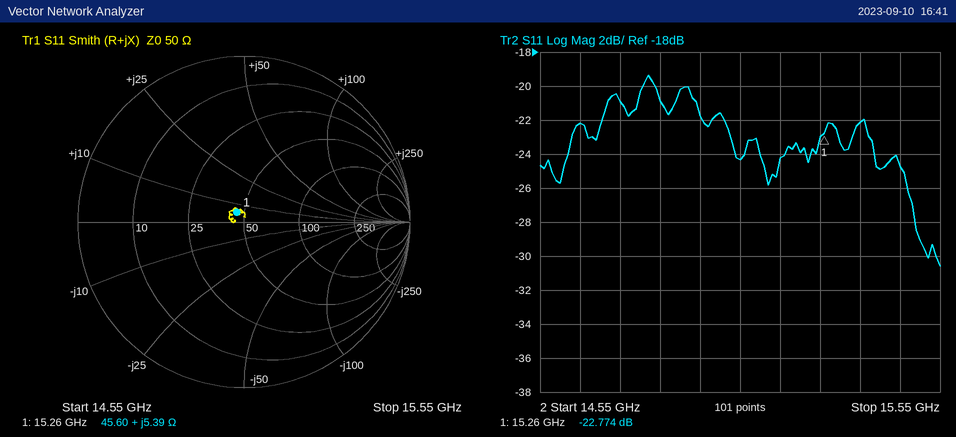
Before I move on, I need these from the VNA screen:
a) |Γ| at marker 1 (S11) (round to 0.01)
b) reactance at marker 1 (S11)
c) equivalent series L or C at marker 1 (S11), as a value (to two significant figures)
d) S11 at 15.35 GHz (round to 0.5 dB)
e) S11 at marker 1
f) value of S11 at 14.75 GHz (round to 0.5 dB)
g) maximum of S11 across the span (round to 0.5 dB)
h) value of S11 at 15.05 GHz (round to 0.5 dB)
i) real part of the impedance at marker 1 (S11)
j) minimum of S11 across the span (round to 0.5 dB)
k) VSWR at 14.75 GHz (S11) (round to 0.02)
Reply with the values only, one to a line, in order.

0.07
+5.39 Ω
56 pH
-22.0 dB
-22.774 dB
-21.0 dB
-19.5 dB
-24.5 dB
45.60 Ω
-30.5 dB
1.20
